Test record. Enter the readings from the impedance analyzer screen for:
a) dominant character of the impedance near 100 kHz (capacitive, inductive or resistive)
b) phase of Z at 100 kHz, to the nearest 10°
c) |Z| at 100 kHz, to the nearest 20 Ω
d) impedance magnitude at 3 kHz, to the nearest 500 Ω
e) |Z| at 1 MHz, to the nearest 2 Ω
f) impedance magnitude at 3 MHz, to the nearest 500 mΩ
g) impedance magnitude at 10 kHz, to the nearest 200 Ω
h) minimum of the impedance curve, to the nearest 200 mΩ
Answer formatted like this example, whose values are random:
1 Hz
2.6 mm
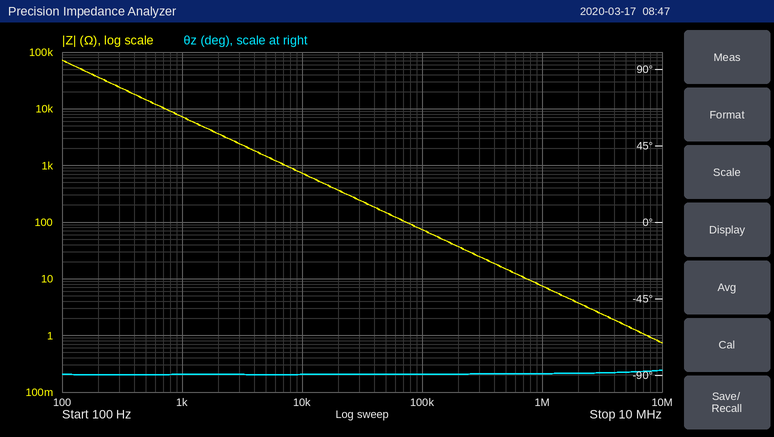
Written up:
capacitive
-90°
80 Ω
2.5 kΩ
8 Ω
2.5 Ω
800 Ω
800 mΩ
